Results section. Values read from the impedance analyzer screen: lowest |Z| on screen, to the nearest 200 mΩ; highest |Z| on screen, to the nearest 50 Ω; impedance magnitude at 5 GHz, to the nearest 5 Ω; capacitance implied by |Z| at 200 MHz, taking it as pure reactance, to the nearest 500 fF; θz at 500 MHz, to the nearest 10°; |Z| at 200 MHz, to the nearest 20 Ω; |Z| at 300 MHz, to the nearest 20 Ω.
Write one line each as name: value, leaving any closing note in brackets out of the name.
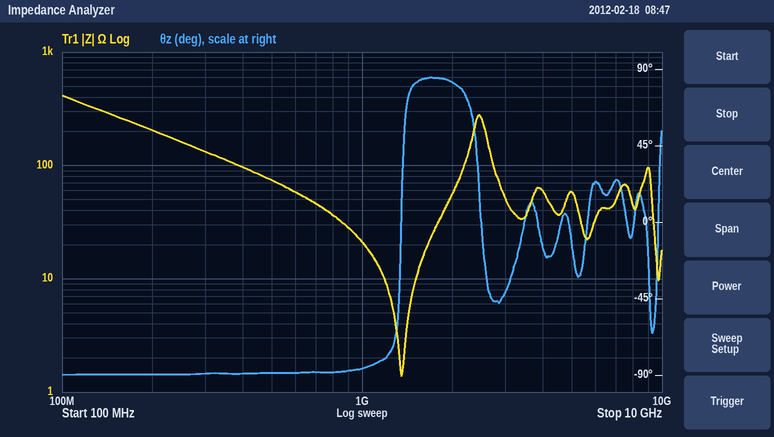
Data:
lowest |Z| on screen, to the nearest 200 mΩ: 1.4 Ω
highest |Z| on screen, to the nearest 50 Ω: 400 Ω
impedance magnitude at 5 GHz, to the nearest 5 Ω: 60 Ω
capacitance implied by |Z| at 200 MHz, taking it as pure reactance, to the nearest 500 fF: 4.0 pF
θz at 500 MHz, to the nearest 10°: -90°
|Z| at 200 MHz, to the nearest 20 Ω: 200 Ω
|Z| at 300 MHz, to the nearest 20 Ω: 140 Ω
